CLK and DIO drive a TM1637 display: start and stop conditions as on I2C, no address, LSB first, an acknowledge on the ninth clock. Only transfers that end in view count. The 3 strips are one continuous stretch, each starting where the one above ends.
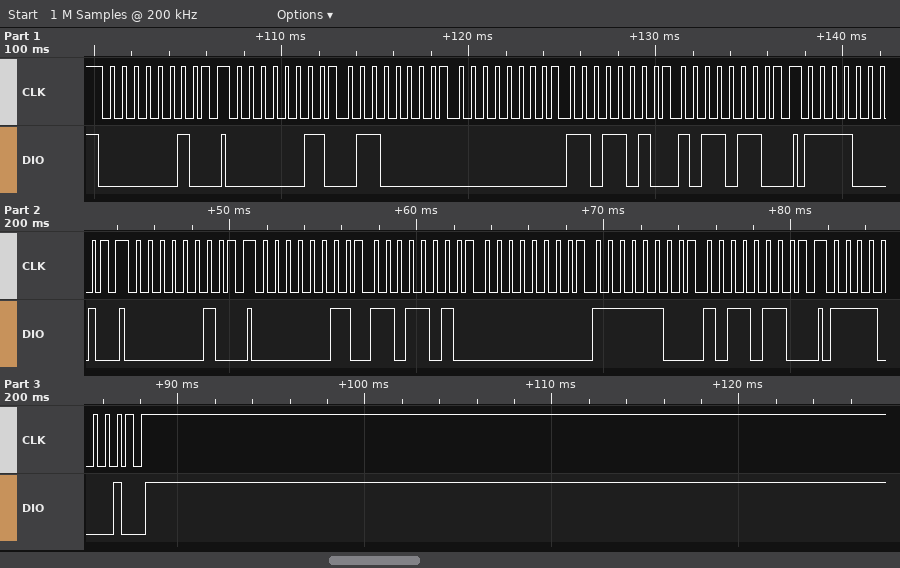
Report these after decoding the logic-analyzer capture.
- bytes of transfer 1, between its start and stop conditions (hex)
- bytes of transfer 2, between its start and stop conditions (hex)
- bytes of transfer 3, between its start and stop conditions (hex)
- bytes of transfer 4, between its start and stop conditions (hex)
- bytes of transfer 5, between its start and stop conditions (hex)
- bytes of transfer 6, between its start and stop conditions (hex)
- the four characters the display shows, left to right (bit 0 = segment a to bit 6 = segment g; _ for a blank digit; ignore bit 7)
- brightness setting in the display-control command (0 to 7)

40
C0 06 00 5B 6D
8F
40
C0 5B 00 3F 6D
8F
2_05
7
